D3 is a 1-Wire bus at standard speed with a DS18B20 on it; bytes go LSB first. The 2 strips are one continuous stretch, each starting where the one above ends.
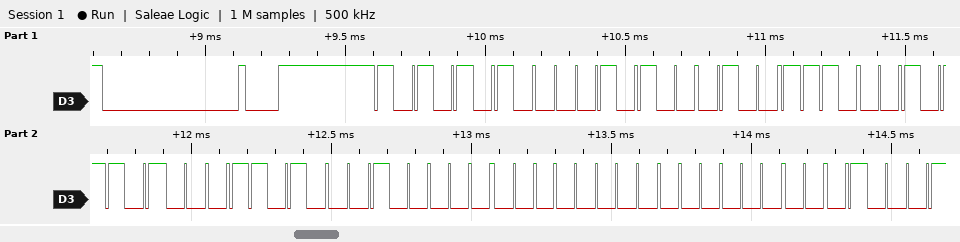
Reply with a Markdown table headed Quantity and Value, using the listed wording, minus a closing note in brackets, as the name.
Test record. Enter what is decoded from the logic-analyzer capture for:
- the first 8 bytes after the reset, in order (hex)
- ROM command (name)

| Quantity | Value |
|---|---|
| the first 8 bytes after the reset, in order | 55 28 72 B4 58 04 00 00 |
| ROM command | Match ROM |
